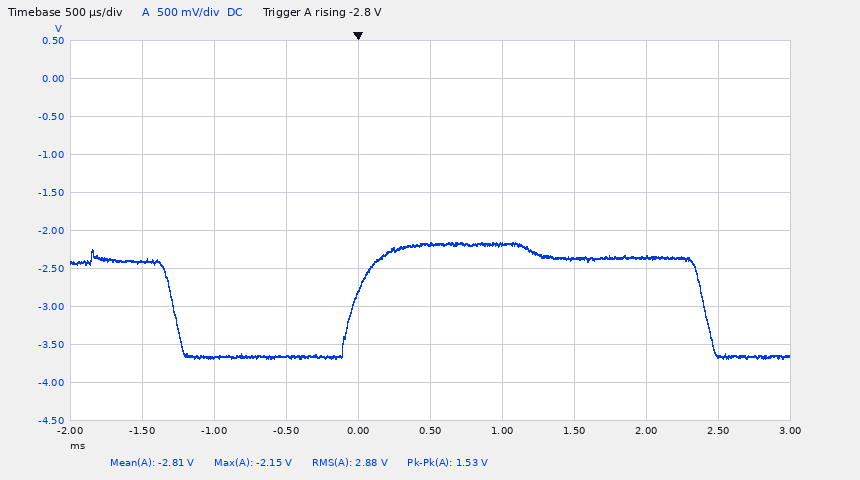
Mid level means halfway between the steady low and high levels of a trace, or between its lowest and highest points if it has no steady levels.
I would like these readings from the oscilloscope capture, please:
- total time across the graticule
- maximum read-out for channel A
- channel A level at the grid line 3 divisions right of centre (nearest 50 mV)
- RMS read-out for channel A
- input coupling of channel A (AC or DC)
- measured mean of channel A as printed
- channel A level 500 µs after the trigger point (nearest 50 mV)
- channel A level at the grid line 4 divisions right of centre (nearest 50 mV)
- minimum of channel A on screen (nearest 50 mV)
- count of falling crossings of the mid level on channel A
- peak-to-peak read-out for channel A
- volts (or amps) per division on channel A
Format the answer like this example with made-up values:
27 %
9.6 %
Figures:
5 ms
-2.15 V
-2.35 V
2.88 V
DC
-2.81 V
-2.20 V
-3.65 V
-3.70 V
2
1.53 V
500 mV
